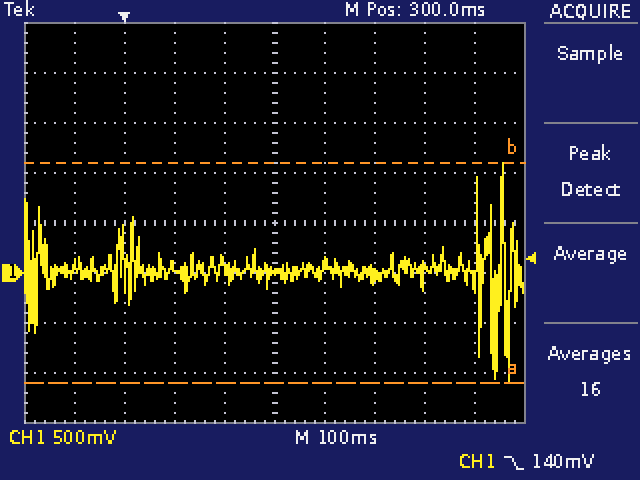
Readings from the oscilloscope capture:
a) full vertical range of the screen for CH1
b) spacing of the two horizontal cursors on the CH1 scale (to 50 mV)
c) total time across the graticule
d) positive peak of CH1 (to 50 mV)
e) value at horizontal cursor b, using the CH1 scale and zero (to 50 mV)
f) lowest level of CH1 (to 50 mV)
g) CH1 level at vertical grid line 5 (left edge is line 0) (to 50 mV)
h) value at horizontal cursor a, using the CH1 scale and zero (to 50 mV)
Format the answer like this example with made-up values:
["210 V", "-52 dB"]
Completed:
["4 V", "2.20 V", "1 s", "1.10 V", "1.10 V", "-1.10 V", "0 mV", "-1.10 V"]
